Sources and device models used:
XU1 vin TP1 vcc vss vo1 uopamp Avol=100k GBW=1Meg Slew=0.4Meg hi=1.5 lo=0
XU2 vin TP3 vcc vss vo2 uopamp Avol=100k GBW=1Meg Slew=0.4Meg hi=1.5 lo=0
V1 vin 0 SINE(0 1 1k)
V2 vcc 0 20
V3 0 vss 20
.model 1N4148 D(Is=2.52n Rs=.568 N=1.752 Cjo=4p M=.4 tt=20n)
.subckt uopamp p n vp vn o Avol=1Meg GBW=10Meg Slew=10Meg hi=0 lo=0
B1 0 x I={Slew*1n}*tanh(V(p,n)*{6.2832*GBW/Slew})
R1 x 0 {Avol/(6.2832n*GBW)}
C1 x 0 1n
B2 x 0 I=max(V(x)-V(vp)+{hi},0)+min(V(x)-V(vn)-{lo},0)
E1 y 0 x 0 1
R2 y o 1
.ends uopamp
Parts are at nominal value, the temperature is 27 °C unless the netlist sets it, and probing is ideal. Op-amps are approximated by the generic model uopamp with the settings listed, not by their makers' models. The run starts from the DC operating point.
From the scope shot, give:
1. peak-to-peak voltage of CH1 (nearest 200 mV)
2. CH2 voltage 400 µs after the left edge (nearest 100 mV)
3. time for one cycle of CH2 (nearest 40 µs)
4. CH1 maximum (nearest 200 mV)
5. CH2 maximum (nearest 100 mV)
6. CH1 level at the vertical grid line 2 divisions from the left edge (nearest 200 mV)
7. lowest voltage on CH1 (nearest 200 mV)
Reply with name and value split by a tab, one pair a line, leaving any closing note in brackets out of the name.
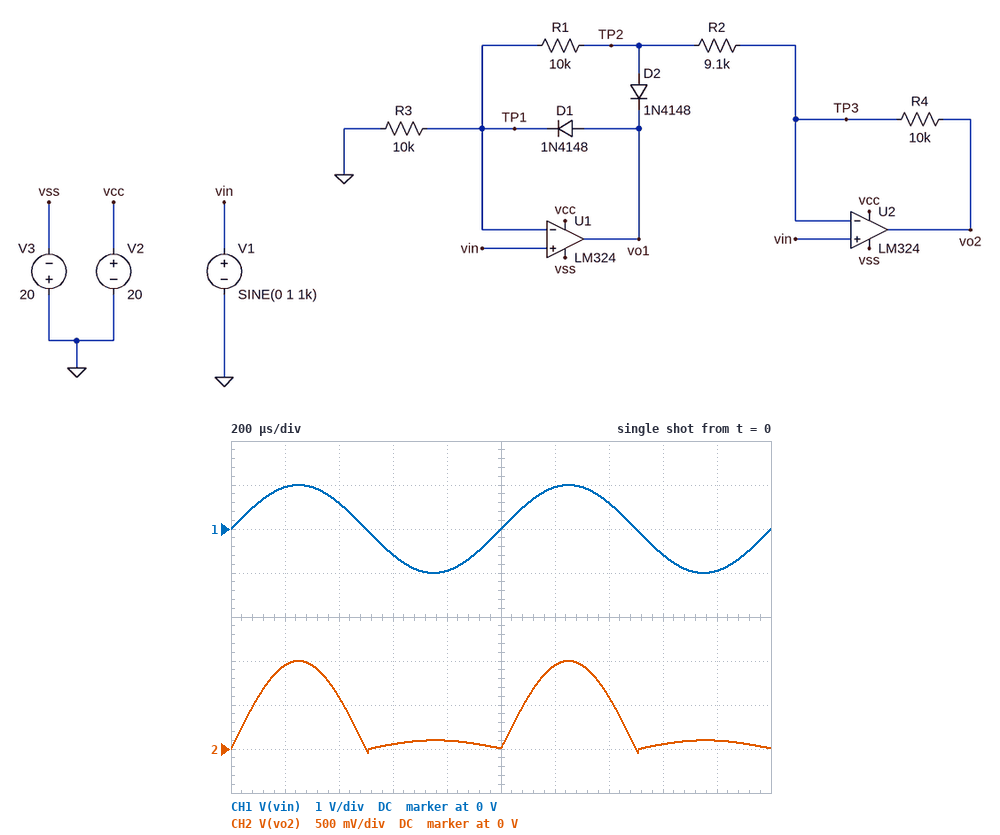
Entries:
peak-to-peak voltage of CH1	2.0 V
CH2 voltage 400 µs after the left edge	600 mV
time for one cycle of CH2	1.00 ms
CH1 maximum	1.0 V
CH2 maximum	1.0 V
CH1 level at the vertical grid line 2 divisions from the left edge	600 mV
lowest voltage on CH1	-1.0 V
